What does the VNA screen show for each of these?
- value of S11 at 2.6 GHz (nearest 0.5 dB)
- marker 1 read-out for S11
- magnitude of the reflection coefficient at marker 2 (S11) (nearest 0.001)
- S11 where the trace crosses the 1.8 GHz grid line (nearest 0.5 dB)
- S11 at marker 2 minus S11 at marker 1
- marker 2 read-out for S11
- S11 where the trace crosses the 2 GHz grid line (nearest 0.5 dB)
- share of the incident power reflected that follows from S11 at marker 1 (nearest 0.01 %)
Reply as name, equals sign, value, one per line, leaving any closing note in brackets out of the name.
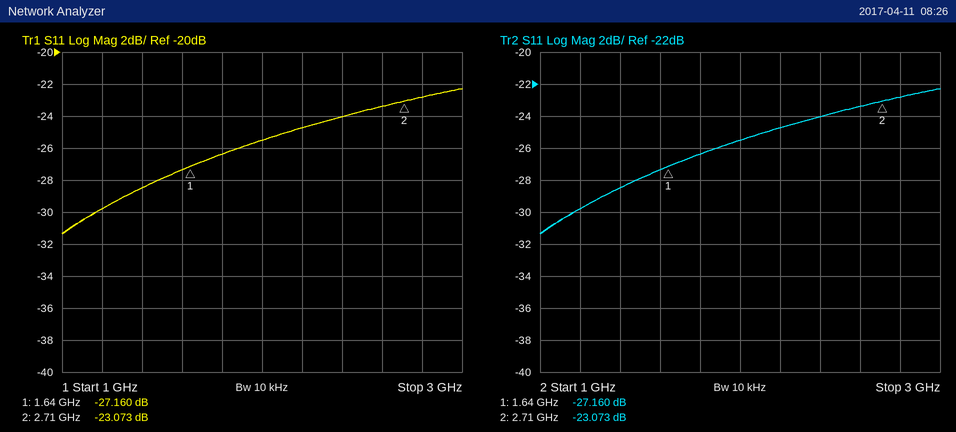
value of S11 at 2.6 GHz = -23.5 dB
marker 1 read-out for S11 = -27.160 dB
magnitude of the reflection coefficient at marker 2 (S11) = 0.070
S11 where the trace crosses the 1.8 GHz grid line = -26.5 dB
S11 at marker 2 minus S11 at marker 1 = 4.087 dB
marker 2 read-out for S11 = -23.073 dB
S11 where the trace crosses the 2 GHz grid line = -25.5 dB
share of the incident power reflected that follows from S11 at marker 1 = 0.19 %
